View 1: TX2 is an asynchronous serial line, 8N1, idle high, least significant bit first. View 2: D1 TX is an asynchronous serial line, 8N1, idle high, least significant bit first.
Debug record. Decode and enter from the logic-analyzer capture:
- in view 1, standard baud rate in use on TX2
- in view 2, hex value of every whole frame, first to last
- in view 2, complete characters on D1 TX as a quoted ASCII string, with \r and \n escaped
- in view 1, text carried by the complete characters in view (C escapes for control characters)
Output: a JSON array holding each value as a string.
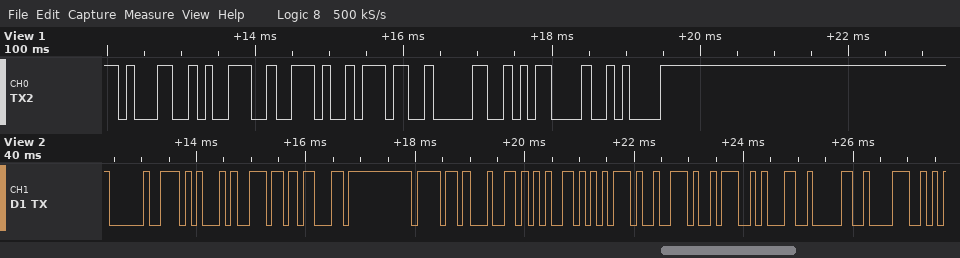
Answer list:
["9600 baud", "20 45 6E 63 6F 64 65 75 72 3A 31 30 38", "\" Encodeur:108\"", "\"19.70\\r\\n\""]
